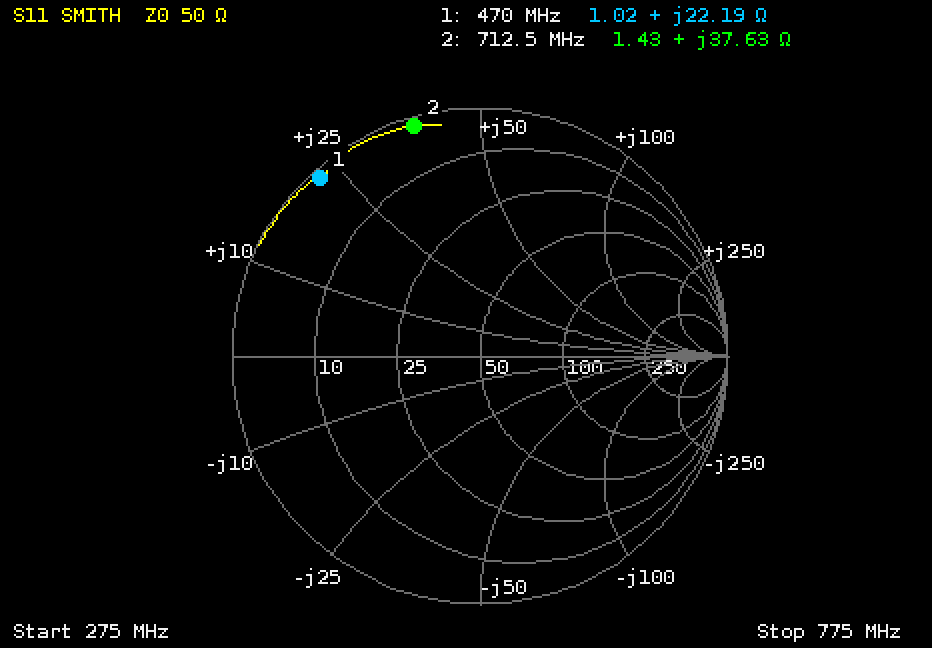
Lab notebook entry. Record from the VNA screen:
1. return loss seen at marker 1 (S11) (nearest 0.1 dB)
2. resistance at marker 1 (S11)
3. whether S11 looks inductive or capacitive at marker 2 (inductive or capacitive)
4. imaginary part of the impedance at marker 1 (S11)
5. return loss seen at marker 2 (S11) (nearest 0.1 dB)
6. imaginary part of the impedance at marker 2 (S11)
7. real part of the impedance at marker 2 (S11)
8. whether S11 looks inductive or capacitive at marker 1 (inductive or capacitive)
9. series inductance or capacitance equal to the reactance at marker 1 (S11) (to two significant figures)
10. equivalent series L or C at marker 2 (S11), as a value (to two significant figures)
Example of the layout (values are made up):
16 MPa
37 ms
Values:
0.3 dB
1.02 Ω
inductive
+22.19 Ω
0.3 dB
+37.63 Ω
1.43 Ω
inductive
7.5 nH
8.4 nH
